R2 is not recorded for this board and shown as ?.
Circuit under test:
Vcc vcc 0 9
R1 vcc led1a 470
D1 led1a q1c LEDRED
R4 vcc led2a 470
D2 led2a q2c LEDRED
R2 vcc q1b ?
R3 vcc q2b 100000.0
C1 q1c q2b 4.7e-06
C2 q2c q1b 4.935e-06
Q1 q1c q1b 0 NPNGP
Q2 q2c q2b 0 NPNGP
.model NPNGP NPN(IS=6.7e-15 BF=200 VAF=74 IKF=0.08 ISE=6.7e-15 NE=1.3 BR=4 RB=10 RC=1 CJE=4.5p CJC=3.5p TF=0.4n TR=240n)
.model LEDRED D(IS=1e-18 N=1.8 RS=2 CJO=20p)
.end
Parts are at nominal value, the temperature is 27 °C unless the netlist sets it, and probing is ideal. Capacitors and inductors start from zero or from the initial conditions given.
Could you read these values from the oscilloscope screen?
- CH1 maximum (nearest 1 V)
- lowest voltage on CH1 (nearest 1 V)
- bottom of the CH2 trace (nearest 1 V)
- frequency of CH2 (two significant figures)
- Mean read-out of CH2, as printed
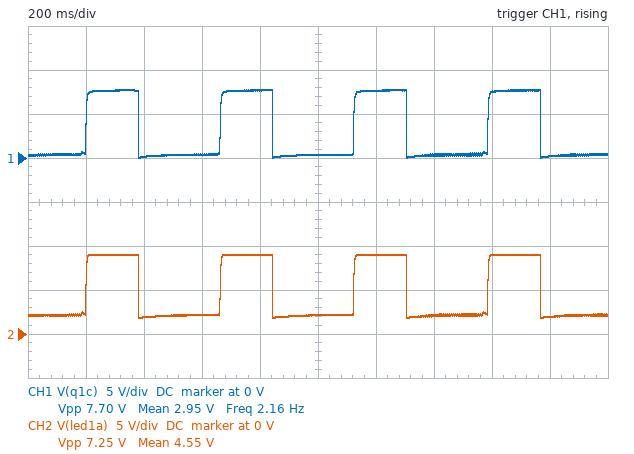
8 V
0 V
2 V
2.2 Hz
4.55 V
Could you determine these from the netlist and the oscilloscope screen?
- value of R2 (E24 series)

75 kΩ
